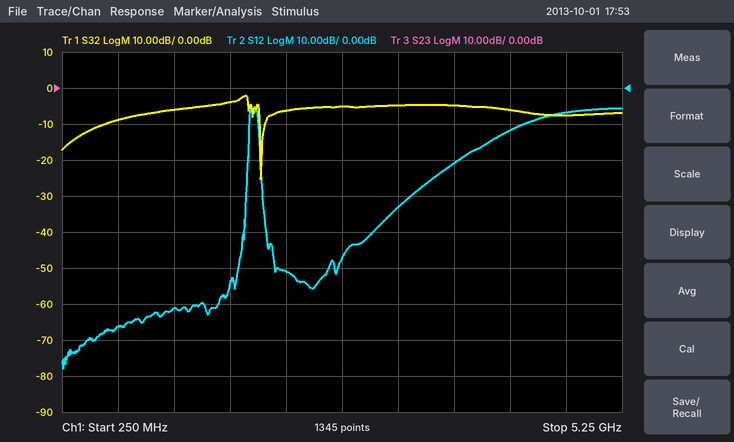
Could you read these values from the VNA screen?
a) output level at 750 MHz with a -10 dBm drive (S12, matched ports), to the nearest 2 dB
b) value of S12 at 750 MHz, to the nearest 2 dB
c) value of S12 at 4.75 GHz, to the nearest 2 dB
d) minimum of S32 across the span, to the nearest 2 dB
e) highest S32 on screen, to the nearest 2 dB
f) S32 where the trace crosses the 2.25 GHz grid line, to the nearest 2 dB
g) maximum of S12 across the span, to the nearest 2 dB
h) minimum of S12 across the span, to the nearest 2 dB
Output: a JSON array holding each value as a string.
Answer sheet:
["-76 dBm", "-66 dB", "-6 dB", "-26 dB", "-2 dB", "-6 dB", "-6 dB", "-78 dB"]
